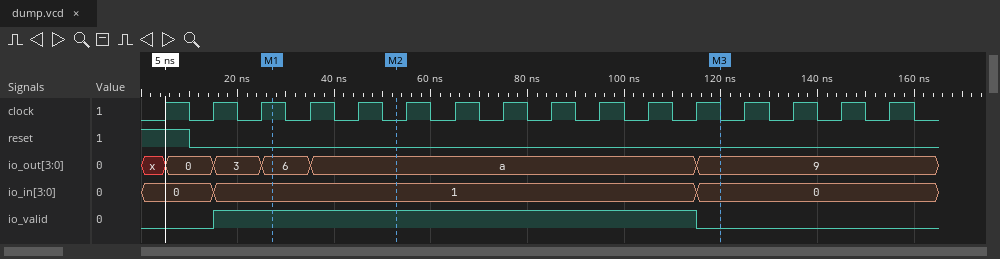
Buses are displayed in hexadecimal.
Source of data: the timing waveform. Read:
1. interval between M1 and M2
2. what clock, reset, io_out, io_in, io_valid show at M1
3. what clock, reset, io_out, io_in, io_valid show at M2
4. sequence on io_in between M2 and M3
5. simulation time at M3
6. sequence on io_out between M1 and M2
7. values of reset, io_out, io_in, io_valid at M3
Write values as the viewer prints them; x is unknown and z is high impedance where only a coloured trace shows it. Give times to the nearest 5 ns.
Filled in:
25 ns
clock=1, reset=0, io_out=6, io_in=1, io_valid=1
clock=0, reset=0, io_out=a, io_in=1, io_valid=1
1, 0
120 ns
6, a
reset=0, io_out=9, io_in=0, io_valid=0
